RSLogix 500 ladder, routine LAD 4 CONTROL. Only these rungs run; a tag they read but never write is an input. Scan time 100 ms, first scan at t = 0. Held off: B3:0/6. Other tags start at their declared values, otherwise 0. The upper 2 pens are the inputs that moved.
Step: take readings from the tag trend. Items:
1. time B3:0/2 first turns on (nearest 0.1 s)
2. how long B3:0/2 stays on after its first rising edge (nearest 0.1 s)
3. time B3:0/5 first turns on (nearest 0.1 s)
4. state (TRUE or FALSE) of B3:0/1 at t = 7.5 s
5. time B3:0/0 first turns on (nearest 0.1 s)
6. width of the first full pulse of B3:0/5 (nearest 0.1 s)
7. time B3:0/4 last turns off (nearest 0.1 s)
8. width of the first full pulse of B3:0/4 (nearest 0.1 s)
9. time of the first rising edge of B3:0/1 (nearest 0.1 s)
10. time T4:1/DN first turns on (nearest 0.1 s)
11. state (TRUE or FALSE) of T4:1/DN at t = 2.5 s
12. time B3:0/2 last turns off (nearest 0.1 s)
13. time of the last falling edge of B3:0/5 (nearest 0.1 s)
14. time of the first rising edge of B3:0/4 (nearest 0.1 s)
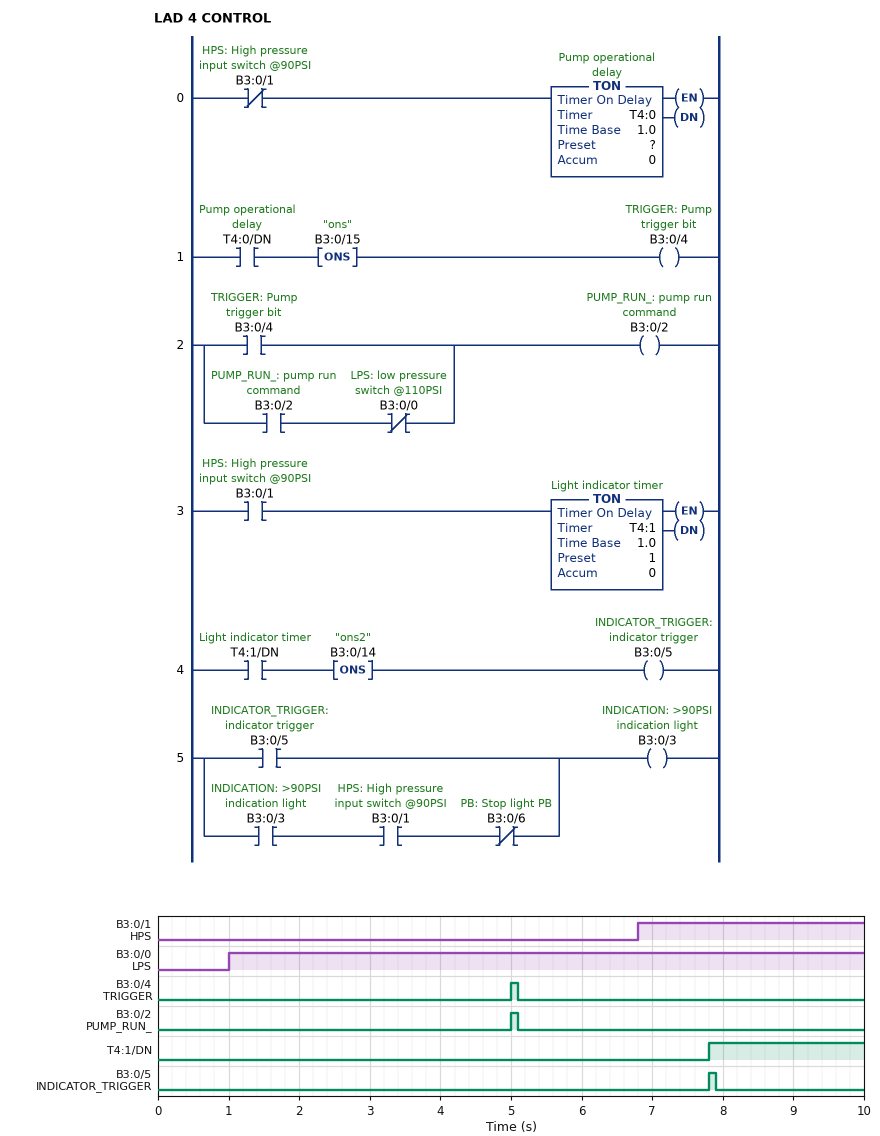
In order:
5.0 s
0.1 s
7.8 s
TRUE
1.0 s
0.1 s
5.1 s
0.1 s
6.8 s
7.8 s
FALSE
5.1 s
7.9 s
5.0 s
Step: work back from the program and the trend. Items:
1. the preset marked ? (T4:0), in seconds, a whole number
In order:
5 s
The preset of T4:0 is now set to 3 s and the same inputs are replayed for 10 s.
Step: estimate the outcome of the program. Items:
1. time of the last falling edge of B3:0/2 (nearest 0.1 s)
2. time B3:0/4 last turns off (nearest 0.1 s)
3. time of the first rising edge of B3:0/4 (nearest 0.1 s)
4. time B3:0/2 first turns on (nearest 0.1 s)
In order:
3.1 s
3.1 s
3.0 s
3.0 s
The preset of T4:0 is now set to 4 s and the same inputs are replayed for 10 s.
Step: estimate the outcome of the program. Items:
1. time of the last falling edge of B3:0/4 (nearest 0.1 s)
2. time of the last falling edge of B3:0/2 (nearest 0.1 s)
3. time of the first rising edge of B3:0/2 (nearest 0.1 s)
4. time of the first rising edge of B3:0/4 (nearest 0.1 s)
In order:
4.1 s
4.1 s
4.0 s
4.0 s
